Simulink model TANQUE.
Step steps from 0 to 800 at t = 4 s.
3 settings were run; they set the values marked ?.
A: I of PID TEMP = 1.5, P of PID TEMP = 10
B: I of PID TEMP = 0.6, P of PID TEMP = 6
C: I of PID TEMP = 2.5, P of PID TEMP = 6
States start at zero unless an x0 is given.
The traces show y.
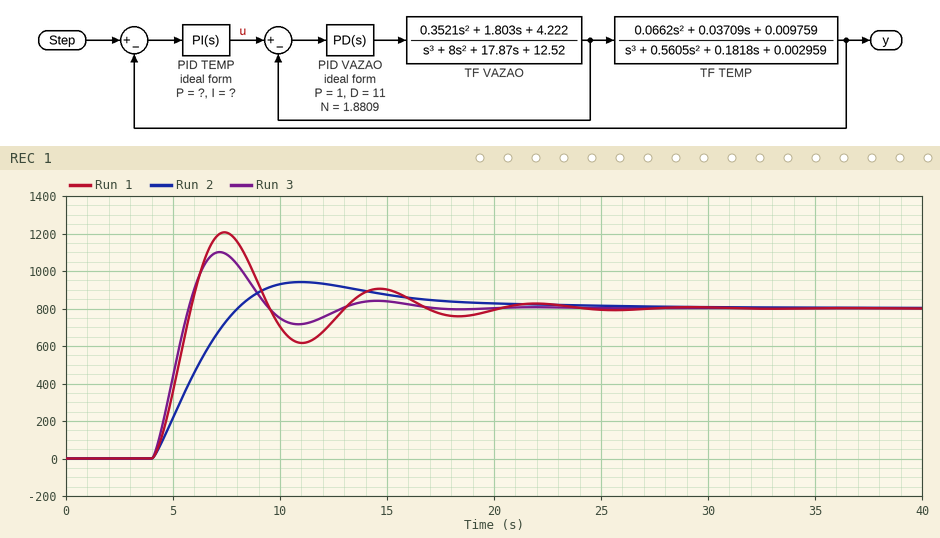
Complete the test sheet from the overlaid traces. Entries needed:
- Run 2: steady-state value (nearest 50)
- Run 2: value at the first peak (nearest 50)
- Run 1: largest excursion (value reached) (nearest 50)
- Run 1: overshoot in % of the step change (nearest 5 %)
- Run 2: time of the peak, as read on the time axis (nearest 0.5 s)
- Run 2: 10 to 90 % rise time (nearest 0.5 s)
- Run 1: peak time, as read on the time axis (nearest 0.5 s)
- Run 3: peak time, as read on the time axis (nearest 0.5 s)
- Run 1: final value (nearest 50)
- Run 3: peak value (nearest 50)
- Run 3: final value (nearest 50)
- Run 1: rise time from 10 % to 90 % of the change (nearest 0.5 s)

800
950
1200
50 %
11.0 s
3.0 s
7.5 s
7.0 s
800
1100
800
1.5 s
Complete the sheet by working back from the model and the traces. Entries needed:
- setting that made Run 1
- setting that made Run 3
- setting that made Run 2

C
A
B
